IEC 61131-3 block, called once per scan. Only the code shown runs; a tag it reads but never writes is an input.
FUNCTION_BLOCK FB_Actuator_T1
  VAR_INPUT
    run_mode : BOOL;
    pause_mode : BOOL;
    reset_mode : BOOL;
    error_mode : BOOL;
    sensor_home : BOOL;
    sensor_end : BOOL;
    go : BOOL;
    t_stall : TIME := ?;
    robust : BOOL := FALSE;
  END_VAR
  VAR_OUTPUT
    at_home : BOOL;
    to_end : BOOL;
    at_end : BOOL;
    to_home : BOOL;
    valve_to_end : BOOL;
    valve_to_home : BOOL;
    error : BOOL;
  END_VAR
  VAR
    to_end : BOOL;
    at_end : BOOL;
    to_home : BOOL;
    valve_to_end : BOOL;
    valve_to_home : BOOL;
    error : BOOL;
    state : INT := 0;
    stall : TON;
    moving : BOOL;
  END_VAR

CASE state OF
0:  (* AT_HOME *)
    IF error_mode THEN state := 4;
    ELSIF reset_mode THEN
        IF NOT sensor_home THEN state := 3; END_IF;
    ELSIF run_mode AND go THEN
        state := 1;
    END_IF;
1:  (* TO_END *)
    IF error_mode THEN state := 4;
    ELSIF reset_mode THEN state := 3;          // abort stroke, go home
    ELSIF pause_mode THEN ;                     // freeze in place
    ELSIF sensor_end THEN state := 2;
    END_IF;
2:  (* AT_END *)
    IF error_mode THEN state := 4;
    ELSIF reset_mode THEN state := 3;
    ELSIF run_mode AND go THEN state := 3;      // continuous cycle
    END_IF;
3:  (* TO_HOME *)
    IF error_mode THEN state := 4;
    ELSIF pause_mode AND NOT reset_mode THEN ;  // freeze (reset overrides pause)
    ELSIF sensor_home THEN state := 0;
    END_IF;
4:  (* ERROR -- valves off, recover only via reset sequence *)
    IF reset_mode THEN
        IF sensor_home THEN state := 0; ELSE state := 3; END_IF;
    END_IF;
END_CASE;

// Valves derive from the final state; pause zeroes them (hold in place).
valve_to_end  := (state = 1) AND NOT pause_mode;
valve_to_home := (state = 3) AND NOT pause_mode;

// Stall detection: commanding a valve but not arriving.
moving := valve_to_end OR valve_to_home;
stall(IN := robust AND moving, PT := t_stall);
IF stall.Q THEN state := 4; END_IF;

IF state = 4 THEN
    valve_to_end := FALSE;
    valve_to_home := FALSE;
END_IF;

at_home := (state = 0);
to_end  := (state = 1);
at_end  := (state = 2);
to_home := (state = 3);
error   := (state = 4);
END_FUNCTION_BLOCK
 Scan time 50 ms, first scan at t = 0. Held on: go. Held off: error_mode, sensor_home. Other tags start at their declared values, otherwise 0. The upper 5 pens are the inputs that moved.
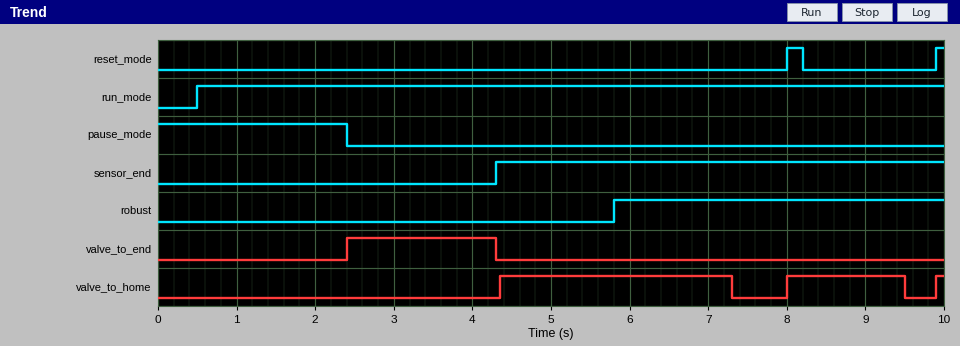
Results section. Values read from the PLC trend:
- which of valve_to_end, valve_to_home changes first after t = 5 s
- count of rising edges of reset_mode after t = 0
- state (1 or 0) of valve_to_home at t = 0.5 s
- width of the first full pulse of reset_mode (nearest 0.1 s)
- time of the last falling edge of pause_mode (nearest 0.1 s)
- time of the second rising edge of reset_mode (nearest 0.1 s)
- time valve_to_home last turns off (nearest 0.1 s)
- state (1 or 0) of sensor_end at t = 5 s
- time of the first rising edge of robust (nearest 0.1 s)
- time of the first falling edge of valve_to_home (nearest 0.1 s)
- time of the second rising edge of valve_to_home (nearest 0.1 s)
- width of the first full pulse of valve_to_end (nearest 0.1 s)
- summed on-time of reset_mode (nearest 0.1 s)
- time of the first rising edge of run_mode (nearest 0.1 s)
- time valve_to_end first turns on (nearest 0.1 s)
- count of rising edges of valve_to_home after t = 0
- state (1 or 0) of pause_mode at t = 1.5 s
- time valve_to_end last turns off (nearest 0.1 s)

valve_to_home
2
0
0.2 s
2.4 s
9.9 s
9.5 s
1
5.8 s
7.3 s
8.0 s
1.9 s
0.3 s
0.5 s
2.4 s
3
1
4.3 s
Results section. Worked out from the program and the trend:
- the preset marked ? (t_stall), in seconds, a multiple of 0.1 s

1.5 s
